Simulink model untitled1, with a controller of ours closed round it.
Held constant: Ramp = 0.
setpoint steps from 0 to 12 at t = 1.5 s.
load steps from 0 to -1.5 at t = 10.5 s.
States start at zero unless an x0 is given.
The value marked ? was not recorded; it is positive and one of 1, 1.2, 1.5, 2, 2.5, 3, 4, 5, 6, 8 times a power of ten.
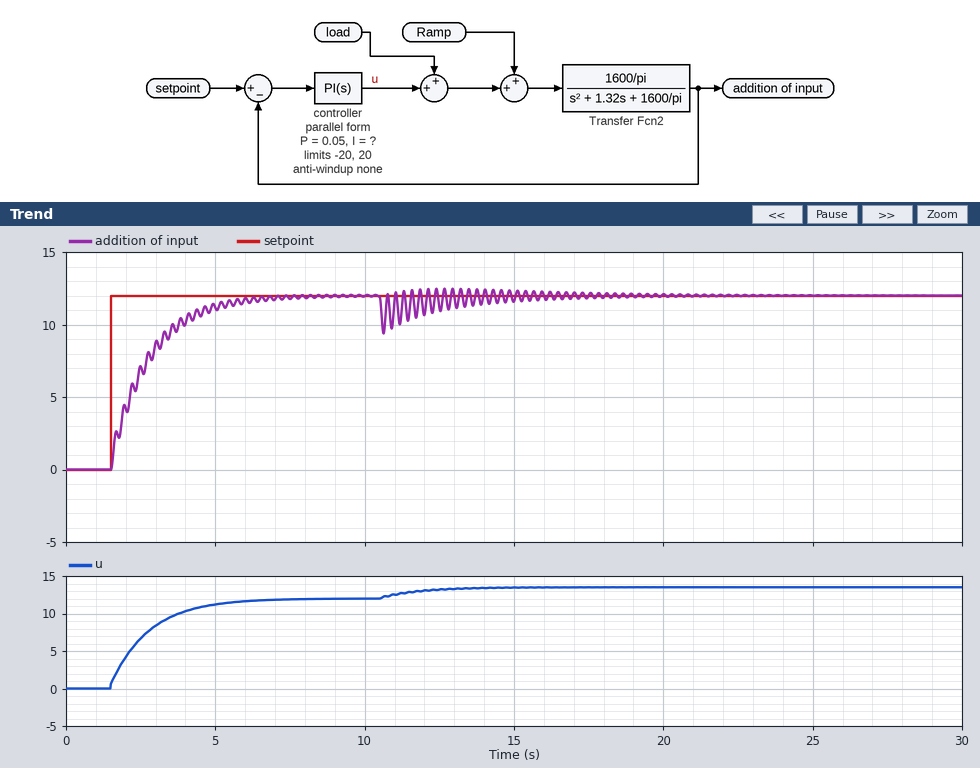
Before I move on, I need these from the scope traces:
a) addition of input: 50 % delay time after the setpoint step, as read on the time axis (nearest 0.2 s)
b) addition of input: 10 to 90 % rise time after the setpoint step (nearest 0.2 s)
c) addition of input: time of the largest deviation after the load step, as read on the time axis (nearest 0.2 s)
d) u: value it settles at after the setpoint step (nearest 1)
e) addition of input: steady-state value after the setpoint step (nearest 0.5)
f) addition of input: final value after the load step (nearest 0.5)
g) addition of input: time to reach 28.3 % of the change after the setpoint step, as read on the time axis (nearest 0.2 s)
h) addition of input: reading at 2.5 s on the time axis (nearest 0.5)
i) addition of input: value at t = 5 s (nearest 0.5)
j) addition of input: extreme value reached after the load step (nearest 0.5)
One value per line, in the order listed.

2.4 s
2.8 s
10.6 s
12
12.0
12.0
1.8 s
7.0
11.0
9.5
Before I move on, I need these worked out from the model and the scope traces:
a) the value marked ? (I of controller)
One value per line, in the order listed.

0.8
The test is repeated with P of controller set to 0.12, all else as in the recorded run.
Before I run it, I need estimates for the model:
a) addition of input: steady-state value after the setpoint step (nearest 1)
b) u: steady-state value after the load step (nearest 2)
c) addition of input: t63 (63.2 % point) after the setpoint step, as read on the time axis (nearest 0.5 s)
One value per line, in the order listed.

12
14
2.5 s
